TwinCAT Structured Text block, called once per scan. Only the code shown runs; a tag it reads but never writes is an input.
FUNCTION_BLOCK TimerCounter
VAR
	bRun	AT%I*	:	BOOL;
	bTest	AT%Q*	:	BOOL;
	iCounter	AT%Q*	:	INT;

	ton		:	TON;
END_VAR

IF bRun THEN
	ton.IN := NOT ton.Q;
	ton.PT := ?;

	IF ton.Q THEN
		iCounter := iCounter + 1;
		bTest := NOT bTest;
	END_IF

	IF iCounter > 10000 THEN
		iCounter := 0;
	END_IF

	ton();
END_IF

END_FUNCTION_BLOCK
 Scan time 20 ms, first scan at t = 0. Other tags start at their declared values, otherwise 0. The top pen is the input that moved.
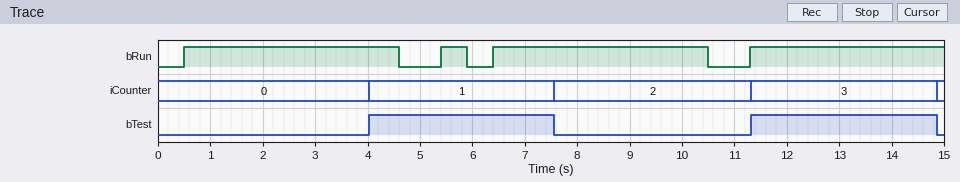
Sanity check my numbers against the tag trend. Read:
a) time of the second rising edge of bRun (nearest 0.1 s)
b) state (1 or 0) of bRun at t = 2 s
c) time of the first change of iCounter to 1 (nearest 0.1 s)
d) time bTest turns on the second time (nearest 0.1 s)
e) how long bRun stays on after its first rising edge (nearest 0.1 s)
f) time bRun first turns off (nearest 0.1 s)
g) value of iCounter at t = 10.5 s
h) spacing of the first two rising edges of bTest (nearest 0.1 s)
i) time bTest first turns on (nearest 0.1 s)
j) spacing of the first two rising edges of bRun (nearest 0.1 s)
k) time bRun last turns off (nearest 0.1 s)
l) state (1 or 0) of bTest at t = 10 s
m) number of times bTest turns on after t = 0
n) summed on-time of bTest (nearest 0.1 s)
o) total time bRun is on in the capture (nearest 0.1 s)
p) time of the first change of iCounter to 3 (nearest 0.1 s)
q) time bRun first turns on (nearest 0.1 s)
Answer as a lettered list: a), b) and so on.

a) 5.4 s
b) 1
c) 4.0 s
d) 11.3 s
e) 4.1 s
f) 4.6 s
g) 2
h) 7.3 s
i) 4.0 s
j) 4.9 s
k) 10.5 s
l) 0
m) 2
n) 7.1 s
o) 12.4 s
p) 11.3 s
q) 0.5 s
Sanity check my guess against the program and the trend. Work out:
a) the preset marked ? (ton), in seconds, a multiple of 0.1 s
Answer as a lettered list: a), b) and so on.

a) 3.5 s
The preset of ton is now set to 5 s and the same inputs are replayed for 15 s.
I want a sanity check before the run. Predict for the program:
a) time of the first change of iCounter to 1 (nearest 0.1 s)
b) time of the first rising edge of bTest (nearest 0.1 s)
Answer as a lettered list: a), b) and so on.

a) 5.5 s
b) 5.5 s
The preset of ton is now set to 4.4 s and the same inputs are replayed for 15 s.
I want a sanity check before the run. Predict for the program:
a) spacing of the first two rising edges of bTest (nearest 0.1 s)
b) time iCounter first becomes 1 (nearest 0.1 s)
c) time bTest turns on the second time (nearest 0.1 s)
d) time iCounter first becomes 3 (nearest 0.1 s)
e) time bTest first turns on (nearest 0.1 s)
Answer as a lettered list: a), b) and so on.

a) 8.9 s
b) 5.4 s
c) 14.3 s
d) 14.3 s
e) 5.4 s
